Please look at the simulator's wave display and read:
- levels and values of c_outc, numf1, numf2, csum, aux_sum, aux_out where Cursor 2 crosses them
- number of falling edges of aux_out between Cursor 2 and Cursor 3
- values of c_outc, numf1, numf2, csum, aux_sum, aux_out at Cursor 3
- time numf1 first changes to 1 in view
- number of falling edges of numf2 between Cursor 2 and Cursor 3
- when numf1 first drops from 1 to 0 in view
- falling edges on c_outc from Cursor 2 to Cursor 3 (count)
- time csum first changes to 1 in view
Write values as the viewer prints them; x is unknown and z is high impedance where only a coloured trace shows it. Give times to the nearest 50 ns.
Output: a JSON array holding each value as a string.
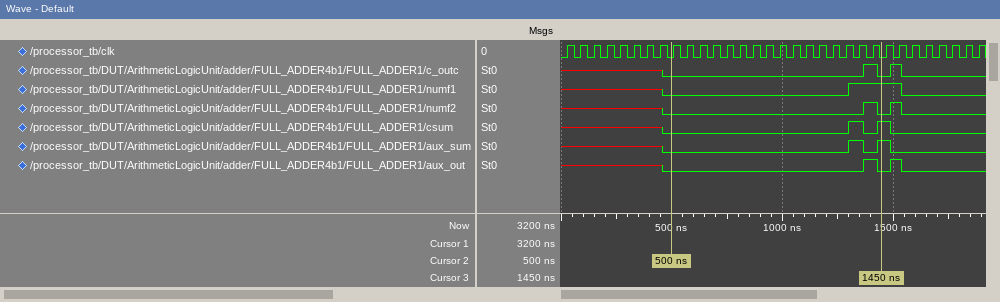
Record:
["c_outc=0, numf1=0, numf2=0, csum=0, aux_sum=0, aux_out=0", "1", "c_outc=0, numf1=1, numf2=0, csum=1, aux_sum=1, aux_out=0", "1300 ns", "1", "1550 ns", "1", "1300 ns"]
